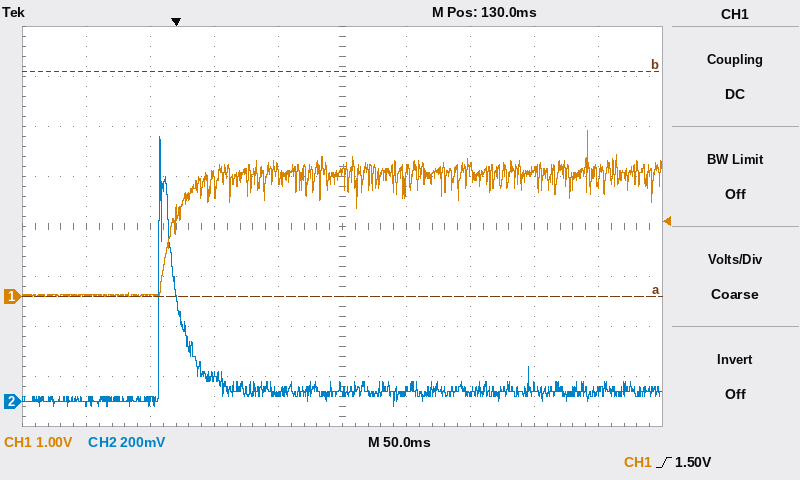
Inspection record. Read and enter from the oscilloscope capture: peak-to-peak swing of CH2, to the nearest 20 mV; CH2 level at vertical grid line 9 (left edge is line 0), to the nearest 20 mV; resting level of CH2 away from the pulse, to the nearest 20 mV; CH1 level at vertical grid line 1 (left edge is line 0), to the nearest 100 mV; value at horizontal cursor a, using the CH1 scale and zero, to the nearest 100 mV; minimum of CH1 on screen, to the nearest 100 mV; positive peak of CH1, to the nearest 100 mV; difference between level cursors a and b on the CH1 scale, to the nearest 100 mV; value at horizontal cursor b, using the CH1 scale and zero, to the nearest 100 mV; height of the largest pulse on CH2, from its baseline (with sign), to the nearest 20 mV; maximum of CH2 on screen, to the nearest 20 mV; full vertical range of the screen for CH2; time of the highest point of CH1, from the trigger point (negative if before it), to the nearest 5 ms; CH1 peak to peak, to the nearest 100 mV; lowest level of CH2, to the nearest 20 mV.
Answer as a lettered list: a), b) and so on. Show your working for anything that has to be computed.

a) 1.06 V − (-20 mV) = 1.08 V
b) 40 mV
c) 40 mV
d) 0.0 V
e) 0.0 V
f) 0.0 V
g) 3.3 V
h) 4.5 V
i) 4.5 V
j) 1.06 V − (40 mV) = +1.02 V
k) 1.06 V
l) 1.6 V
m) +320 ms
n) 3.3 V − (0.0 V) = 3.3 V
o) -20 mV
